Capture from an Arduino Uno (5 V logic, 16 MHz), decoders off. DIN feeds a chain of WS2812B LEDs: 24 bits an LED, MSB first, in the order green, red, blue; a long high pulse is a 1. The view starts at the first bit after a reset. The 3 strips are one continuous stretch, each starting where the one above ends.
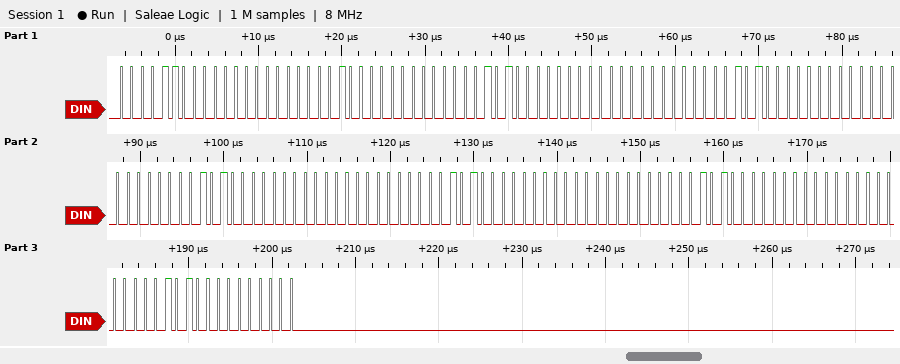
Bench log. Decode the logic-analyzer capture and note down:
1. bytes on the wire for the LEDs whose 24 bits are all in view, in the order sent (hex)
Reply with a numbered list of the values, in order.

1. 0C 00 04 00 14 00 00 14 00 00 14 00 00 14 00 00 14 00 00 14 00
